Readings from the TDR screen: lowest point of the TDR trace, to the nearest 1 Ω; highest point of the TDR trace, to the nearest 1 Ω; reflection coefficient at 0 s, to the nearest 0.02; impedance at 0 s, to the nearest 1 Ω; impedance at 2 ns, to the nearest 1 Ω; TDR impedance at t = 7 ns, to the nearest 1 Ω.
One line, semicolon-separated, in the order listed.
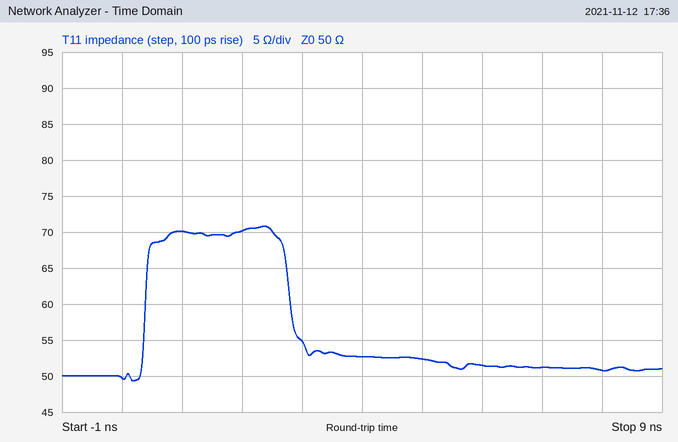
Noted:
49 Ω; 71 Ω; 0.00; 50 Ω; 70 Ω; 51 Ω
